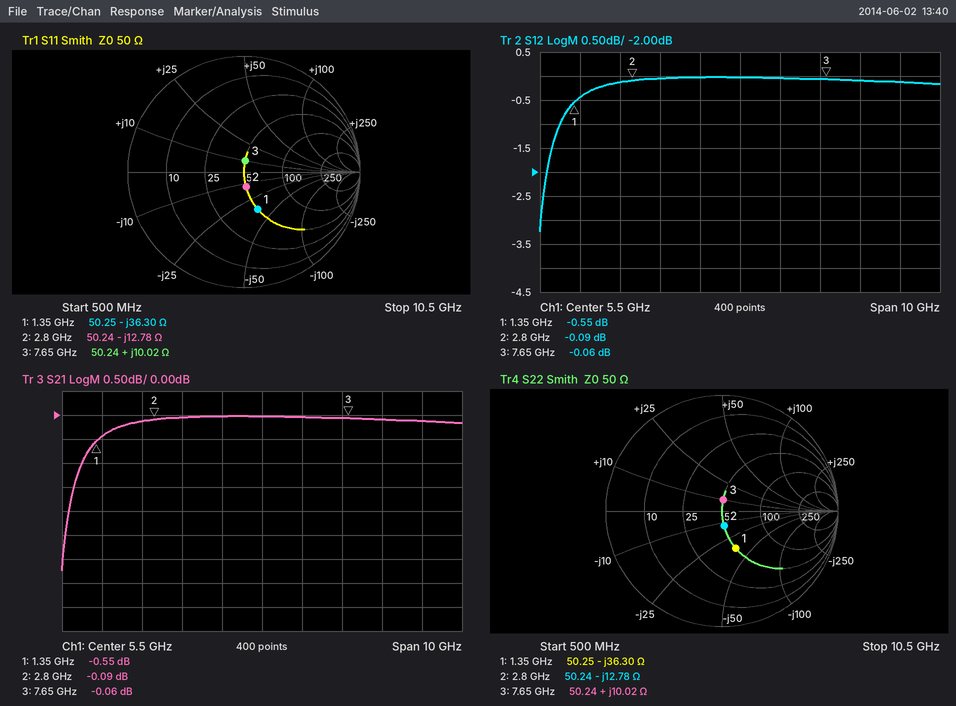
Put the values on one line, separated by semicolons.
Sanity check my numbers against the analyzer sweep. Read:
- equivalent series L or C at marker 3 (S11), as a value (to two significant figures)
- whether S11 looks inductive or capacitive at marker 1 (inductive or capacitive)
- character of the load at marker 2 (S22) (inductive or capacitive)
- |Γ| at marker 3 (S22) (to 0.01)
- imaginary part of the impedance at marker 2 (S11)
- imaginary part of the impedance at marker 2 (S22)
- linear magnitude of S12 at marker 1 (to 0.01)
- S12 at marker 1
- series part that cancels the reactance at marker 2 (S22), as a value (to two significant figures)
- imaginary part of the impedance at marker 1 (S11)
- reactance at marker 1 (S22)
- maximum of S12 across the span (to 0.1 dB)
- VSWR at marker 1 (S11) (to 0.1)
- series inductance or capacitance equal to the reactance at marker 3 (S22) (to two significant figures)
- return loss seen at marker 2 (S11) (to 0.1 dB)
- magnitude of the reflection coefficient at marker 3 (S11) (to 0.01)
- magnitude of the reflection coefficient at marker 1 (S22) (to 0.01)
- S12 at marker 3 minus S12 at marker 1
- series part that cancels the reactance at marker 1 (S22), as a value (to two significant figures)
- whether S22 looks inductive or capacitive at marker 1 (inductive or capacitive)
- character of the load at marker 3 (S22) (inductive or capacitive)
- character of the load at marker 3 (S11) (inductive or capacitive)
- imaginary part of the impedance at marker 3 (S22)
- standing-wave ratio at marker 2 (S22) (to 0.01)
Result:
210 pH; capacitive; capacitive; 0.10; -12.78 Ω; -12.78 Ω; 0.94; -0.55 dB; 730 pH; -36.30 Ω; -36.30 Ω; 0.0 dB; 2.0; 210 pH; 18.0 dB; 0.10; 0.34; 0.49 dB; 4.3 nH; capacitive; inductive; inductive; +10.02 Ω; 1.29
